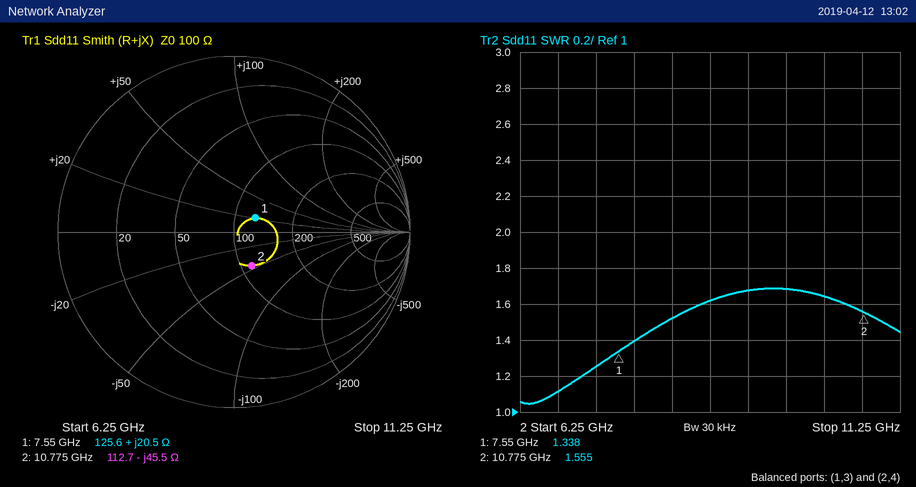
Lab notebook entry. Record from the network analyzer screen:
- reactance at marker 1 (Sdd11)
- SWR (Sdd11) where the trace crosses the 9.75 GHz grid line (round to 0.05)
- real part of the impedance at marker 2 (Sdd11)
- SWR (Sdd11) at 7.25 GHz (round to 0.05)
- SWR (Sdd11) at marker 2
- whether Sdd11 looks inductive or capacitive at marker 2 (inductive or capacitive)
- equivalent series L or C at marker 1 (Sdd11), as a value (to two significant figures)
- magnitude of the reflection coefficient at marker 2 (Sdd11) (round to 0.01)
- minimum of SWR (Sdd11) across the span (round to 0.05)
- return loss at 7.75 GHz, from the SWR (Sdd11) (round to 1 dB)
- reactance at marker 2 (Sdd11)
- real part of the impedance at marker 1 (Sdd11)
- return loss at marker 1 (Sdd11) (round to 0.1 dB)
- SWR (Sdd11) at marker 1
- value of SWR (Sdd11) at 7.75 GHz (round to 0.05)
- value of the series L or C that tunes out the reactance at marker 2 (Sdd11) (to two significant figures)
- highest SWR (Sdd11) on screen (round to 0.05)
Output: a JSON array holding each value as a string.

["+20.5 Ω", "1.70", "112.7 Ω", "1.25", "1.555", "capacitive", "430 pH", "0.22", "1.05", "16 dB", "-45.5 Ω", "125.6 Ω", "16.8 dB", "1.338", "1.40", "670 pH", "1.70"]
